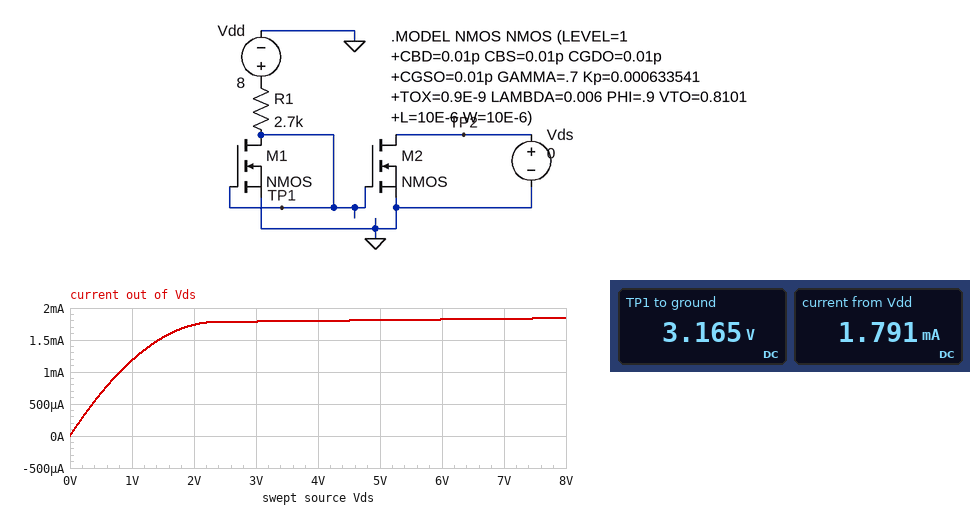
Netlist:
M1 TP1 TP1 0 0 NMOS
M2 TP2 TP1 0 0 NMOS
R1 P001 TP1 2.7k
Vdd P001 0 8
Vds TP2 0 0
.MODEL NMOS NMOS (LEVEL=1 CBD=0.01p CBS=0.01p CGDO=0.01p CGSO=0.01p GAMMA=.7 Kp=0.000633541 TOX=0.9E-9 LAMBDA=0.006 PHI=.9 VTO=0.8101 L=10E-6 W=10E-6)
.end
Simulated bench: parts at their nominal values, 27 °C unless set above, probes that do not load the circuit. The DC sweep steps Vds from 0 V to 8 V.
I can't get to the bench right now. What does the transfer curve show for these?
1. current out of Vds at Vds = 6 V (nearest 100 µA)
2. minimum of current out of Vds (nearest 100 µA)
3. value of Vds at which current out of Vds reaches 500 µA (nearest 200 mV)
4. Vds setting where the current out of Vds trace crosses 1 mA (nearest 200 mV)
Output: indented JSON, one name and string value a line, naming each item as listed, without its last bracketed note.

{
  "current out of Vds at Vds = 6 V": "1.8 mA",
  "minimum of current out of Vds": "0 A",
  "value of Vds at which current out of Vds reaches 500 µA": "400 mV",
  "Vds setting where the current out of Vds trace crosses 1 mA": "800 mV"
}
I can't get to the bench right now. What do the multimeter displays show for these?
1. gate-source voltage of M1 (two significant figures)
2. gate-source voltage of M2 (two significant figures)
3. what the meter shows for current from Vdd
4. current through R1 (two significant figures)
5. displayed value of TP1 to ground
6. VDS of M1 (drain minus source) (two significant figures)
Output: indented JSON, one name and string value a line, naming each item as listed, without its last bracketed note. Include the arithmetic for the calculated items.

{
  "gate-source voltage of M1": "3.165 V = 3.2 V",
  "gate-source voltage of M2": "3.165 V = 3.2 V",
  "what the meter shows for current from Vdd": "1.791 mA",
  "current through R1": "(8 V - 3.165 V) / 2.7 kΩ = 1.8 mA",
  "displayed value of TP1 to ground": "3.165 V",
  "VDS of M1 (drain minus source)": "3.165 V = 3.2 V"
}
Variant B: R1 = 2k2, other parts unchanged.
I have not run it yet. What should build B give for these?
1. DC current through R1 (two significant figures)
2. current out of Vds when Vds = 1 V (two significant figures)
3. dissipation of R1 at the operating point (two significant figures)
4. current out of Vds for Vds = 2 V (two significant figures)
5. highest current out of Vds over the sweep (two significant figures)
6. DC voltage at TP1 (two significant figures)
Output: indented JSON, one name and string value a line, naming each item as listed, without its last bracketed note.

{
  "DC current through R1": "2.1 mA",
  "current out of Vds when Vds = 1 V": "1.3 mA",
  "dissipation of R1 at the operating point": "9.8 mW",
  "current out of Vds for Vds = 2 V": "2.0 mA",
  "highest current out of Vds over the sweep": "2.2 mA",
  "DC voltage at TP1": "3.4 V"
}
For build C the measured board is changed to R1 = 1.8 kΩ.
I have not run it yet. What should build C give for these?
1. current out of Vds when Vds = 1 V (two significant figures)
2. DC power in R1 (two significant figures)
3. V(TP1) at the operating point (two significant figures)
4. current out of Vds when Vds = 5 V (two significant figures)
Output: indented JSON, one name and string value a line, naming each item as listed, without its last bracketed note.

{
  "current out of Vds when Vds = 1 V": "1.4 mA",
  "DC power in R1": "11 mW",
  "V(TP1) at the operating point": "3.6 V",
  "current out of Vds when Vds = 5 V": "2.5 mA"
}
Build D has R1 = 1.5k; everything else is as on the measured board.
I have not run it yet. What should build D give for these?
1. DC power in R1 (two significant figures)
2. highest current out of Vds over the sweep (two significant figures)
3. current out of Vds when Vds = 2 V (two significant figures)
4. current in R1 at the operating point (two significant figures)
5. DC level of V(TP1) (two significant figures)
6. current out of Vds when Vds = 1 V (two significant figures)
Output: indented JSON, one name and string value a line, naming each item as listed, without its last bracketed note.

{
  "DC power in R1": "12 mW",
  "highest current out of Vds over the sweep": "2.9 mA",
  "current out of Vds when Vds = 2 V": "2.5 mA",
  "current in R1 at the operating point": "2.8 mA",
  "DC level of V(TP1)": "3.8 V",
  "current out of Vds when Vds = 1 V": "1.6 mA"
}
